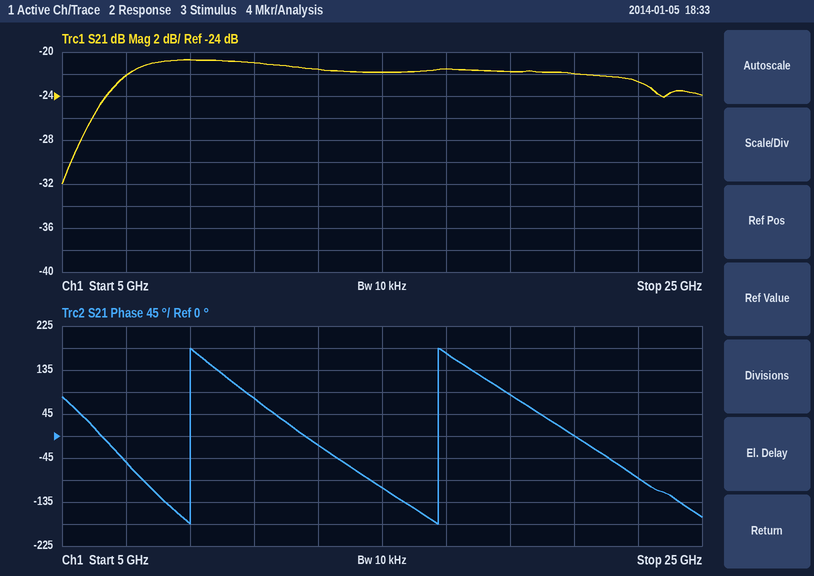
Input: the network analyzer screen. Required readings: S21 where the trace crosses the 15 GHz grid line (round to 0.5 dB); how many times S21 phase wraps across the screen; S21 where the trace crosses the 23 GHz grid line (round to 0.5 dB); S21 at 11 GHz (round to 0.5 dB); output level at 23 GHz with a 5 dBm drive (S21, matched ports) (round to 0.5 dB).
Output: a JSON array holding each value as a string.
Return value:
["-22.0 dB", "2", "-22.5 dB", "-21.0 dB", "-17.5 dBm"]
